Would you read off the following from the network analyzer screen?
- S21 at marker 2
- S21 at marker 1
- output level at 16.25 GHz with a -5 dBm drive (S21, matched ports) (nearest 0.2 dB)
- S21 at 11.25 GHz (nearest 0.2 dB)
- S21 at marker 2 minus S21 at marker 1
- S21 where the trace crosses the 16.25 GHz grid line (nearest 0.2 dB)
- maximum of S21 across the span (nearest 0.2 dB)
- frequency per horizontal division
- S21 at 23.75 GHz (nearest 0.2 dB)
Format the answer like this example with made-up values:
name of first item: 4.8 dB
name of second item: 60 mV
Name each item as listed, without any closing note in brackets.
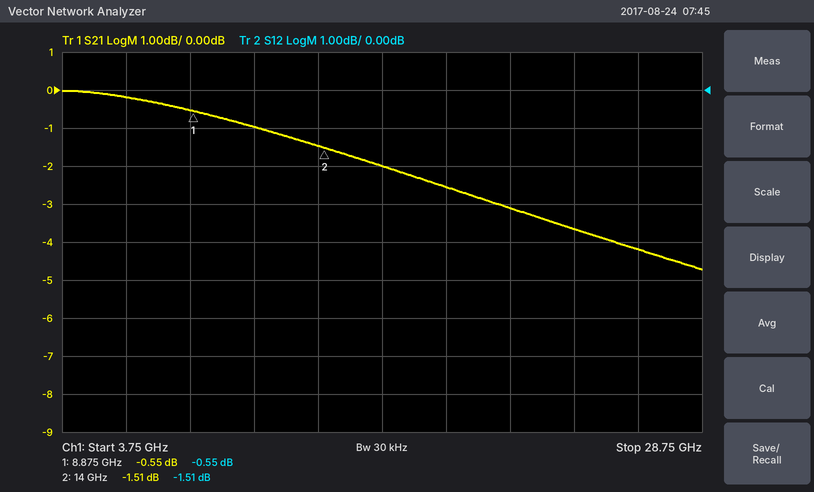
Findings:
S21 at marker 2: -1.51 dB
S21 at marker 1: -0.55 dB
output level at 16.25 GHz with a -5 dBm drive (S21, matched ports): -7.0 dBm
S21 at 11.25 GHz: -1.0 dB
S21 at marker 2 minus S21 at marker 1: -0.96 dB
S21 where the trace crosses the 16.25 GHz grid line: -2.0 dB
maximum of S21 across the span: 0.0 dB
frequency per horizontal division: 2.5 GHz
S21 at 23.75 GHz: -3.6 dB
